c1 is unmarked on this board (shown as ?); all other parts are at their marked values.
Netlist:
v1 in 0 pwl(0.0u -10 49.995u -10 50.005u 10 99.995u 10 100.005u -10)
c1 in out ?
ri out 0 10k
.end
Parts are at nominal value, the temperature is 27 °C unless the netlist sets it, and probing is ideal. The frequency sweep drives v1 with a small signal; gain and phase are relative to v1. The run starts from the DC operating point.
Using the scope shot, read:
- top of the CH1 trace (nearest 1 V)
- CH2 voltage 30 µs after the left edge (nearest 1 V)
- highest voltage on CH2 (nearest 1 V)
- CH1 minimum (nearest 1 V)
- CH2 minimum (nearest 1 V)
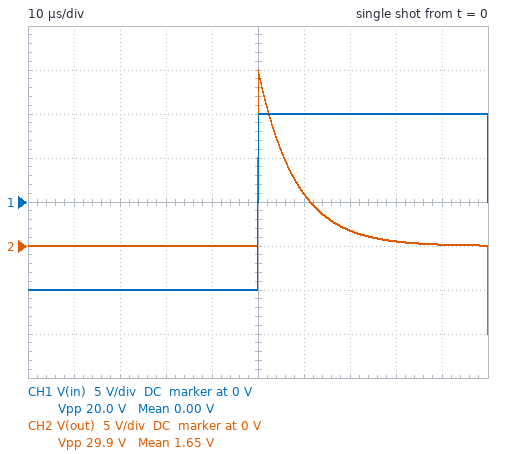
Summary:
10 V
0 V
20 V
-10 V
-10 V
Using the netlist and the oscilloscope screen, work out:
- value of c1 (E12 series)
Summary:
820 pF
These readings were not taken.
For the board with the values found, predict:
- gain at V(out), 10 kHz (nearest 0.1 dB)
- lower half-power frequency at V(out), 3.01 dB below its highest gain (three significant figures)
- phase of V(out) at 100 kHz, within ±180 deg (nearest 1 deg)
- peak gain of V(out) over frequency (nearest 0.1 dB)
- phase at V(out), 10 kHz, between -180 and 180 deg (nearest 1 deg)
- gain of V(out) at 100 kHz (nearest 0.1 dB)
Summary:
-6.8 dB
19.4 kHz
11 deg
0 dB
63 deg
-0.2 dB
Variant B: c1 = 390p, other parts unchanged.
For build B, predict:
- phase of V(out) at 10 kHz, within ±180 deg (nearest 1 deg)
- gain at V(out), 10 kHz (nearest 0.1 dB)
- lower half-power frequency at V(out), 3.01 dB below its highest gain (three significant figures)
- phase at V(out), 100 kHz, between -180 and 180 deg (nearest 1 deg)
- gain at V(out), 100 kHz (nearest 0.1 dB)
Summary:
76 deg
-12.5 dB
40.8 kHz
22 deg
-0.7 dB
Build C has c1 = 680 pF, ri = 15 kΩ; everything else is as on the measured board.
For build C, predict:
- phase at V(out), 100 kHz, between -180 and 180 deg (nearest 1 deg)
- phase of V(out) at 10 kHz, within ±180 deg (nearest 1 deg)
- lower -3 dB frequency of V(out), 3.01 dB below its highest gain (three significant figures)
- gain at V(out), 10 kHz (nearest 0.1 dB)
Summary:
9 deg
57 deg
15.6 kHz
-5.4 dB
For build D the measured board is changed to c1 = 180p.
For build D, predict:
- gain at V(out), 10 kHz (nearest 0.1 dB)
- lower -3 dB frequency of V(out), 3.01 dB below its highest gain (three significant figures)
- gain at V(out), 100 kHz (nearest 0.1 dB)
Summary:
-19.0 dB
88.4 kHz
-2.5 dB
